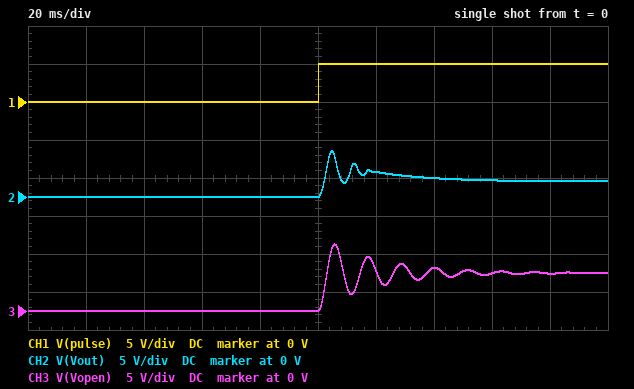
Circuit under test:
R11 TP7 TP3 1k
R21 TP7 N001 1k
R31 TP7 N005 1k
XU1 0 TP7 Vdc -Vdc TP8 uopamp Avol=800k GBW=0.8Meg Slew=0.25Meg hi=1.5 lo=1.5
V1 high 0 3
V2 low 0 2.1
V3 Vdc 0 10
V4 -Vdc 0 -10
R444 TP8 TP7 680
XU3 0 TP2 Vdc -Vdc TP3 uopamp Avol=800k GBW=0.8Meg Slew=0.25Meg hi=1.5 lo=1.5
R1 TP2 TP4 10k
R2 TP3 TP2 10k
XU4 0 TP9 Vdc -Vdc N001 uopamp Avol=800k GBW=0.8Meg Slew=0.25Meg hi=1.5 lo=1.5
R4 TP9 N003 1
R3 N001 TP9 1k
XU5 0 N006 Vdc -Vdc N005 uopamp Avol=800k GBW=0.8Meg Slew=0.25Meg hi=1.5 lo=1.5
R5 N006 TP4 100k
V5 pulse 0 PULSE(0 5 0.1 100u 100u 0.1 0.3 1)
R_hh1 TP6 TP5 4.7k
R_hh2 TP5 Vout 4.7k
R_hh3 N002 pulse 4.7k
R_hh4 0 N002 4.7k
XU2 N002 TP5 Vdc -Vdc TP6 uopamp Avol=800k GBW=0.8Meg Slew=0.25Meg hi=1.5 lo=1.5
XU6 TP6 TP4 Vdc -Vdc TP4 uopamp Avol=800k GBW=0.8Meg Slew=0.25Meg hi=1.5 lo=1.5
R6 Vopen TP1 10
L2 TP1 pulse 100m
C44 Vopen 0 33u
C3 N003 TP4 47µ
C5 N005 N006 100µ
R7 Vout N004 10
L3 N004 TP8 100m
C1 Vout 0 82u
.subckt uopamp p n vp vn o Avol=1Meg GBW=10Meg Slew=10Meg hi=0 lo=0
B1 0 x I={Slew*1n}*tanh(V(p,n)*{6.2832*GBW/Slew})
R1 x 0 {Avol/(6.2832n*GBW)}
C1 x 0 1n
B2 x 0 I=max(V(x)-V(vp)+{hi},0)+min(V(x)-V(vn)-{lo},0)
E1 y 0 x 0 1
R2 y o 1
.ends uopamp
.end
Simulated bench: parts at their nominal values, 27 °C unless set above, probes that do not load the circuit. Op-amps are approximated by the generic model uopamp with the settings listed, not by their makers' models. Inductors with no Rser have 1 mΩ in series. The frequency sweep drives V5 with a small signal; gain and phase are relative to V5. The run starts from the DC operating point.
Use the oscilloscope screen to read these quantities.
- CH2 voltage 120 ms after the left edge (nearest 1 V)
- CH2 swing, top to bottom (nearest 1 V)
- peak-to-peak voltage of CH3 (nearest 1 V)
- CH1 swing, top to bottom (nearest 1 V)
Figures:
3 V
6 V
9 V
5 V
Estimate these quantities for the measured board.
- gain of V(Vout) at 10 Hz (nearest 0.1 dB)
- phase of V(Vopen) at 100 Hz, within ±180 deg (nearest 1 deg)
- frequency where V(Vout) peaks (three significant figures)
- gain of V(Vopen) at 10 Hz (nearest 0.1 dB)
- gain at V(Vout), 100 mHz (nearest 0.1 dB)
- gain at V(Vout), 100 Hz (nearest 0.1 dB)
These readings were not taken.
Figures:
-1.9 dB
-146 deg
1.60 kHz
0.1 dB
-7.8 dB
-0.2 dB
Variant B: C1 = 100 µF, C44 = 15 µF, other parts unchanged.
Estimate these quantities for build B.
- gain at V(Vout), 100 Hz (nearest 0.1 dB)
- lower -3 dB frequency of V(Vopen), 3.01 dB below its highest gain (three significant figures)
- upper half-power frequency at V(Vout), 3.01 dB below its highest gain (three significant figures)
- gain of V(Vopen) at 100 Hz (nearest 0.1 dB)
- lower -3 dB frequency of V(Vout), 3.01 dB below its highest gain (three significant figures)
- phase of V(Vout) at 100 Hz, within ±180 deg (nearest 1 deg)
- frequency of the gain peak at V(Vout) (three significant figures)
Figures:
-0.3 dB
121 Hz
1.70 kHz
7.6 dB
1.42 kHz
-8 deg
1.58 kHz
